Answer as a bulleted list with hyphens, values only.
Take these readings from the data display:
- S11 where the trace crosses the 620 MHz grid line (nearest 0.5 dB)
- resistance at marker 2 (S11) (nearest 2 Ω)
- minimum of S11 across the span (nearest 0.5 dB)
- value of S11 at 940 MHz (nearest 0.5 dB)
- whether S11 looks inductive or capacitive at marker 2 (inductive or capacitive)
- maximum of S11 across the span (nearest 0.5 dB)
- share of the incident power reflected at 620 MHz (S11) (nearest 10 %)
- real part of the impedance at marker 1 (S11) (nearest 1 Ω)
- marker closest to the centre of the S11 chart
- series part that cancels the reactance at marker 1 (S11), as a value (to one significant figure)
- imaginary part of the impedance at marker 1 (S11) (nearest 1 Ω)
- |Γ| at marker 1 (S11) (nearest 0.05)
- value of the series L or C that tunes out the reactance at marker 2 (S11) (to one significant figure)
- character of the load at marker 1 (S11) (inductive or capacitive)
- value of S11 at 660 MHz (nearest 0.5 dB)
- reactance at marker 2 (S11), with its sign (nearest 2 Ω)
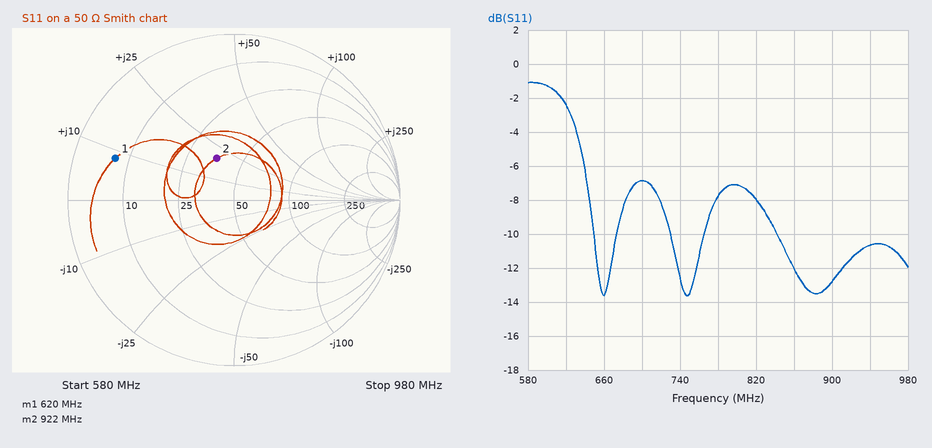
- -2.5 dB
- 36 Ω
- -13.5 dB
- -10.5 dB
- inductive
- -1.0 dB
- 60 %
- 7 Ω
- marker 2
- 30 pF
- +8 Ω
- 0.75
- 9 pF
- inductive
- -13.5 dB
- +20 Ω
